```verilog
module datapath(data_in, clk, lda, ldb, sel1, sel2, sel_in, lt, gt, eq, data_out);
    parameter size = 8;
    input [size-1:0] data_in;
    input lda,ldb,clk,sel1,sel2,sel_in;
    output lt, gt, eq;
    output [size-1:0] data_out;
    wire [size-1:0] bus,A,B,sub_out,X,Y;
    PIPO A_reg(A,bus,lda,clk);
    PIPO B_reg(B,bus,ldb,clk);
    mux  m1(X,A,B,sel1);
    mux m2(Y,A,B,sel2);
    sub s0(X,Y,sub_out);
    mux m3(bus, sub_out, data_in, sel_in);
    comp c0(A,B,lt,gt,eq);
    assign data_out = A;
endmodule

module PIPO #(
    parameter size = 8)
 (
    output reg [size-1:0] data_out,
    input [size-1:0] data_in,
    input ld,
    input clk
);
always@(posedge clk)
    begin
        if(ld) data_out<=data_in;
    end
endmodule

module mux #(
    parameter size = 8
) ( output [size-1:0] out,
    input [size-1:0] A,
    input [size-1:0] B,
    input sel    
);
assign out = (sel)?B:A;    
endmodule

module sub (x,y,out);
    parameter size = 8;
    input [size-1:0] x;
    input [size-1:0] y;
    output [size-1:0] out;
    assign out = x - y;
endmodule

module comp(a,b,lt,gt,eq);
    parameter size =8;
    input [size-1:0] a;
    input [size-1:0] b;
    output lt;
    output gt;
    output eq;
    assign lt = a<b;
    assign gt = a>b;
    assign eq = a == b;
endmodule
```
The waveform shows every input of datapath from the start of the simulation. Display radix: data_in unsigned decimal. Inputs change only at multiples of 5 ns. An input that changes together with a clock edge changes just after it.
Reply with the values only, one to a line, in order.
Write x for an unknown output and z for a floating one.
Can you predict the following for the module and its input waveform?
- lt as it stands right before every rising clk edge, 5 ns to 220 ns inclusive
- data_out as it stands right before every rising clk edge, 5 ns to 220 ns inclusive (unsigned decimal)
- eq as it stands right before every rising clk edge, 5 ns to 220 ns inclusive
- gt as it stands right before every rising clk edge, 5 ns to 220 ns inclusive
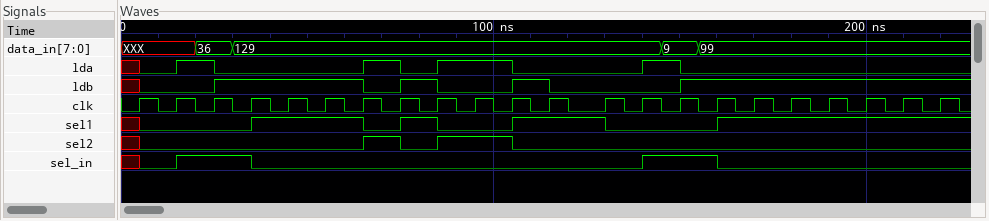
x x x x 1 1 1 0 1 0 0 1 0 0 0 0 1 1 1 1 1 1
x, x, x, 36, 36, 36, 36, 36, 15, 15, 9, 3, 3, 3, 3, 9, 9, 9, 9, 9, 9, 9
x x x x 0 0 0 0 0 0 0 0 1 1 1 0 0 0 0 0 0 0
x x x x 0 0 0 1 0 1 1 0 0 0 0 1 0 0 0 0 0 0
